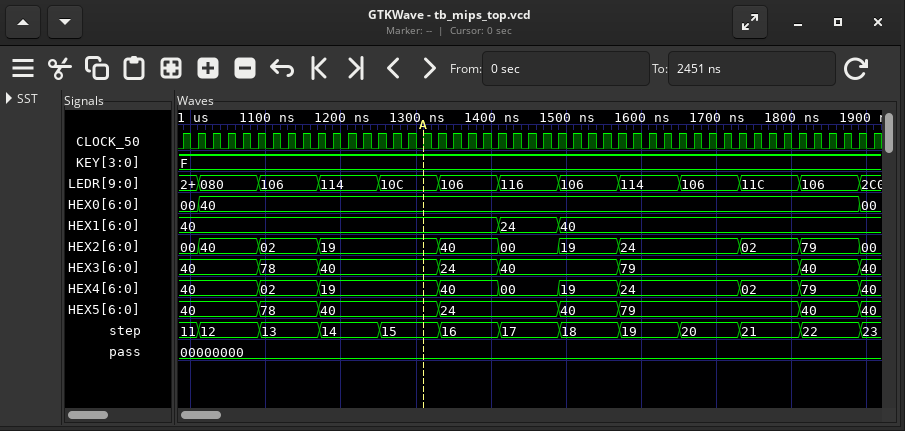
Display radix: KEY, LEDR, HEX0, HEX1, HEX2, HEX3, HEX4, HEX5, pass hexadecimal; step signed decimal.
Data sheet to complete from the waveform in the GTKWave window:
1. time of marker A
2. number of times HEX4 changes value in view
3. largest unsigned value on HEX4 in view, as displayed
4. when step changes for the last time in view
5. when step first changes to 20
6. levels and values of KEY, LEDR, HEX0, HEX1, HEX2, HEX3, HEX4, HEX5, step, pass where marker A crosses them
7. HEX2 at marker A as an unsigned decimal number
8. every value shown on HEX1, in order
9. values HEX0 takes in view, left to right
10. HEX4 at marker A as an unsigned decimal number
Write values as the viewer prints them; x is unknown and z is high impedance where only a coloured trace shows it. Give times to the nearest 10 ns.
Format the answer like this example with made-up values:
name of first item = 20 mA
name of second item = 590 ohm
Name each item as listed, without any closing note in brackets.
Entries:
time of marker A = 1310 ns
number of times HEX4 changes value in view = 9
largest unsigned value on HEX4 in view, as displayed = 79
when step changes for the last time in view = 1890 ns
when step first changes to 20 = 1650 ns
levels and values of KEY, LEDR, HEX0, HEX1, HEX2, HEX3, HEX4, HEX5, step, pass where marker A crosses them = KEY=F, LEDR=10C, HEX0=40, HEX1=40, HEX2=19, HEX3=40, HEX4=19, HEX5=40, step=15, pass=00000000
HEX2 at marker A as an unsigned decimal number = 25
every value shown on HEX1, in order = 40, 24, 40
values HEX0 takes in view, left to right = 00, 40, 00
HEX4 at marker A as an unsigned decimal number = 25
